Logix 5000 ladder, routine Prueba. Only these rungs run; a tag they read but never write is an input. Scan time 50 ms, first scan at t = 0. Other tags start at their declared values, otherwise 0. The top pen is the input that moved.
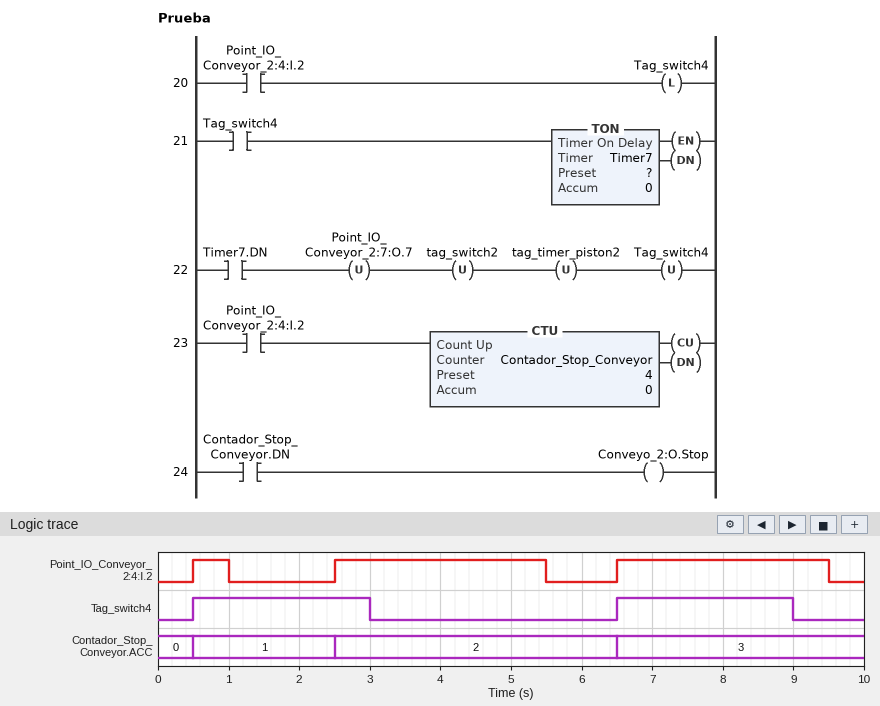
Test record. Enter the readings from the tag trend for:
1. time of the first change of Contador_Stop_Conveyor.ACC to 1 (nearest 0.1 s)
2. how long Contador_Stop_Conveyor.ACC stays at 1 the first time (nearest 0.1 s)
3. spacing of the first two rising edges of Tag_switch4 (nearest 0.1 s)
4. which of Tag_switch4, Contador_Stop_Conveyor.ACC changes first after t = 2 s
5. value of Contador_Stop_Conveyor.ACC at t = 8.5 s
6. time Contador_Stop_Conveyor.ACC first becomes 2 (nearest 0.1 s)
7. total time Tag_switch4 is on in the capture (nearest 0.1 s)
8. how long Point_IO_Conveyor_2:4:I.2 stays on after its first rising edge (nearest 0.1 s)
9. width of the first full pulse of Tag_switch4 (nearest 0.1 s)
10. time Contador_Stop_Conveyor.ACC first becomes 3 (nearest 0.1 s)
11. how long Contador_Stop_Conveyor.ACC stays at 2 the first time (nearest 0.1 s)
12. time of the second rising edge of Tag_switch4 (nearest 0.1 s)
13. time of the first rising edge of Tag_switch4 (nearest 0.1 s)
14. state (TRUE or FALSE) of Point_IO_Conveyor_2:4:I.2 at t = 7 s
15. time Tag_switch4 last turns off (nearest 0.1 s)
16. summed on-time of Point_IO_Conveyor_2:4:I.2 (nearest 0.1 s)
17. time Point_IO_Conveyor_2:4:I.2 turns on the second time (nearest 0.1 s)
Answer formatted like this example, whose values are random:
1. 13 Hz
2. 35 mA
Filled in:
1. 0.5 s
2. 2.0 s
3. 6.0 s
4. Contador_Stop_Conveyor.ACC
5. 3
6. 2.5 s
7. 5.0 s
8. 0.5 s
9. 2.5 s
10. 6.5 s
11. 4.0 s
12. 6.5 s
13. 0.5 s
14. TRUE
15. 9.0 s
16. 6.5 s
17. 2.5 s
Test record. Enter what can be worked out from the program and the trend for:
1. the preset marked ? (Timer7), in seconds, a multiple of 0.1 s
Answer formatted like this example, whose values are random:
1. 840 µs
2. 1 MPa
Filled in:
1. 2.5 s
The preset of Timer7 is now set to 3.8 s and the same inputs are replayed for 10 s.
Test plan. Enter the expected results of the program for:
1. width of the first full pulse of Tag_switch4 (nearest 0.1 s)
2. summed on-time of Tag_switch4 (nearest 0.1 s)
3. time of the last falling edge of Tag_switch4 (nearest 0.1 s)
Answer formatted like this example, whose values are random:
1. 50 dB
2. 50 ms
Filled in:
1. 3.8 s
2. 7.3 s
3. 4.3 s
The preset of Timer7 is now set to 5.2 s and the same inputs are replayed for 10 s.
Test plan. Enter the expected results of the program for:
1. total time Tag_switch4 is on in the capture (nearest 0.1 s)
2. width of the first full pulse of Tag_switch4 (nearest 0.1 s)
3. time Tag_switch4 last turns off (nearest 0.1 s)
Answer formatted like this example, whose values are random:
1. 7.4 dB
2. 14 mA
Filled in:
1. 8.7 s
2. 5.2 s
3. 5.7 s
